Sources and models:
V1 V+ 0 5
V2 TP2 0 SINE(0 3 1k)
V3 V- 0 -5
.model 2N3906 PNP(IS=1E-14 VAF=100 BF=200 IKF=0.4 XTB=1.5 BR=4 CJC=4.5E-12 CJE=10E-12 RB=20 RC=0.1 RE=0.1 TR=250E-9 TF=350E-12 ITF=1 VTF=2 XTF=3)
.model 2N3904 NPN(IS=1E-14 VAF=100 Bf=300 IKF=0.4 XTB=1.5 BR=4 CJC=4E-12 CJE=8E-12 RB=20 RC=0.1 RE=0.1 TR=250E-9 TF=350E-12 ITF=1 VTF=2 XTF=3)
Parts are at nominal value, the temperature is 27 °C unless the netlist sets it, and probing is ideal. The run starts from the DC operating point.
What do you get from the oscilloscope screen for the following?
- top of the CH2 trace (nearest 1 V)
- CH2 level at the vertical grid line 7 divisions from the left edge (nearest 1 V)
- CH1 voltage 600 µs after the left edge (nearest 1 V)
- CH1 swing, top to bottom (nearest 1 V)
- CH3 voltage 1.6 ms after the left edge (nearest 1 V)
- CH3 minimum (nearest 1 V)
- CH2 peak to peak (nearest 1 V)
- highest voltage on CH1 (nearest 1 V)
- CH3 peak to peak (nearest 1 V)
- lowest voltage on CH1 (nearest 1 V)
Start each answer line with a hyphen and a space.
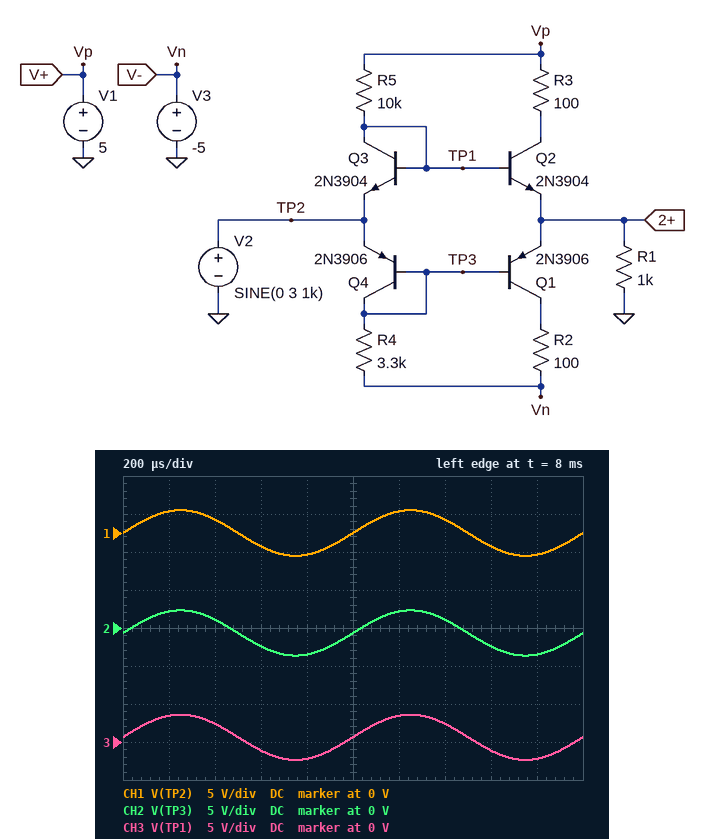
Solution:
- 2 V
- 1 V
- -2 V
- 6 V
- -1 V
- -2 V
- 6 V
- 3 V
- 6 V
- -3 V
